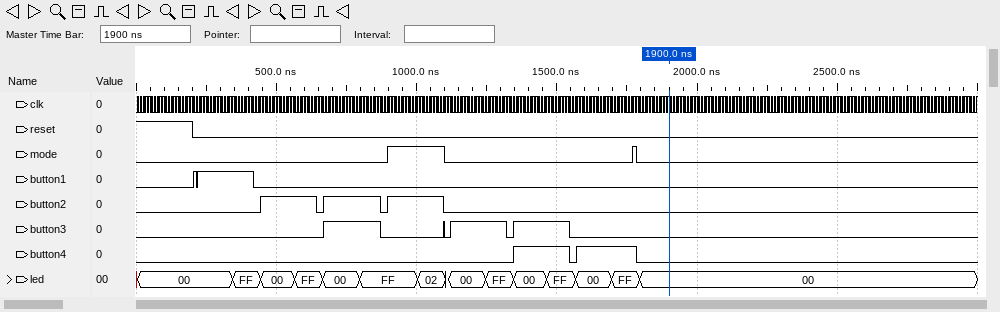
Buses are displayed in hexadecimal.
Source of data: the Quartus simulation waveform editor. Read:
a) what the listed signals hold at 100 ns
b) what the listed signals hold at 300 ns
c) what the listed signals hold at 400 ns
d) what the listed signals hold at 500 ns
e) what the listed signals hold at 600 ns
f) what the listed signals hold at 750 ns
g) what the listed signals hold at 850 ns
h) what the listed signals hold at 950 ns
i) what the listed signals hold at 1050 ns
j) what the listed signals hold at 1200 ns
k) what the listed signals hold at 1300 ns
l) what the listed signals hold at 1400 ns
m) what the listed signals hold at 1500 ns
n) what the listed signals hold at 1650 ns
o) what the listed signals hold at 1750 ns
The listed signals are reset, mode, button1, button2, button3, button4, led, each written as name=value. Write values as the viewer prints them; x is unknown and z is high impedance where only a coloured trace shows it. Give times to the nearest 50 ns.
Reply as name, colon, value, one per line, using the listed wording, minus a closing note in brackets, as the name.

what the listed signals hold at 100 ns: reset=1, mode=0, button1=0, button2=0, button3=0, button4=0, led=00
what the listed signals hold at 300 ns: reset=0, mode=0, button1=1, button2=0, button3=0, button4=0, led=00
what the listed signals hold at 400 ns: reset=0, mode=0, button1=1, button2=0, button3=0, button4=0, led=FF
what the listed signals hold at 500 ns: reset=0, mode=0, button1=0, button2=1, button3=0, button4=0, led=00
what the listed signals hold at 600 ns: reset=0, mode=0, button1=0, button2=1, button3=0, button4=0, led=FF
what the listed signals hold at 750 ns: reset=0, mode=0, button1=0, button2=1, button3=1, button4=0, led=00
what the listed signals hold at 850 ns: reset=0, mode=0, button1=0, button2=1, button3=1, button4=0, led=FF
what the listed signals hold at 950 ns: reset=0, mode=1, button1=0, button2=1, button3=0, button4=0, led=FF
what the listed signals hold at 1050 ns: reset=0, mode=1, button1=0, button2=1, button3=0, button4=0, led=02
what the listed signals hold at 1200 ns: reset=0, mode=0, button1=0, button2=0, button3=1, button4=0, led=00
what the listed signals hold at 1300 ns: reset=0, mode=0, button1=0, button2=0, button3=1, button4=0, led=FF
what the listed signals hold at 1400 ns: reset=0, mode=0, button1=0, button2=0, button3=1, button4=1, led=00
what the listed signals hold at 1500 ns: reset=0, mode=0, button1=0, button2=0, button3=1, button4=1, led=FF
what the listed signals hold at 1650 ns: reset=0, mode=0, button1=0, button2=0, button3=0, button4=1, led=00
what the listed signals hold at 1750 ns: reset=0, mode=0, button1=0, button2=0, button3=0, button4=1, led=FF
